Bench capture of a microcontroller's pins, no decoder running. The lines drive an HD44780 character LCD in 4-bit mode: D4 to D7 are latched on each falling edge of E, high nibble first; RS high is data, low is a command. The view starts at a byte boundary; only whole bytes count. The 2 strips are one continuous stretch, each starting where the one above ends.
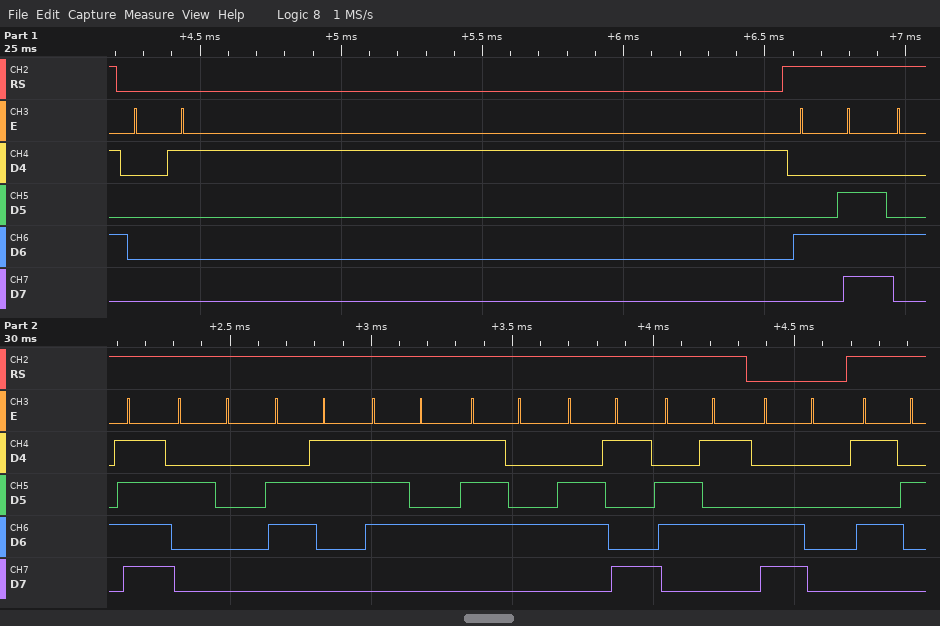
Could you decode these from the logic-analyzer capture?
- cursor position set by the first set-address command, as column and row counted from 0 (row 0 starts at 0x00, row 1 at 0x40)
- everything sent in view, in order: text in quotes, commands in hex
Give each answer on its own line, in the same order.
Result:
column 0, row 1
0x01 "NO cutie" 0xC0 "R"
